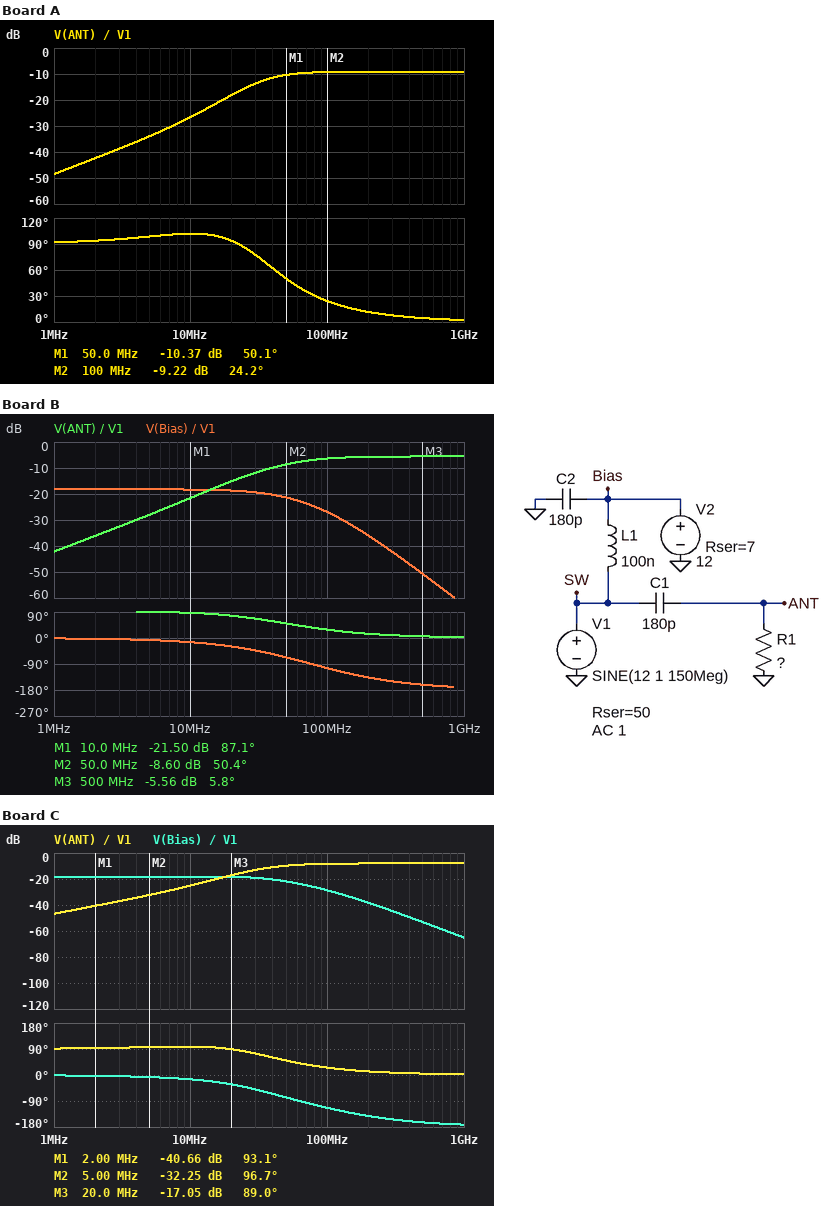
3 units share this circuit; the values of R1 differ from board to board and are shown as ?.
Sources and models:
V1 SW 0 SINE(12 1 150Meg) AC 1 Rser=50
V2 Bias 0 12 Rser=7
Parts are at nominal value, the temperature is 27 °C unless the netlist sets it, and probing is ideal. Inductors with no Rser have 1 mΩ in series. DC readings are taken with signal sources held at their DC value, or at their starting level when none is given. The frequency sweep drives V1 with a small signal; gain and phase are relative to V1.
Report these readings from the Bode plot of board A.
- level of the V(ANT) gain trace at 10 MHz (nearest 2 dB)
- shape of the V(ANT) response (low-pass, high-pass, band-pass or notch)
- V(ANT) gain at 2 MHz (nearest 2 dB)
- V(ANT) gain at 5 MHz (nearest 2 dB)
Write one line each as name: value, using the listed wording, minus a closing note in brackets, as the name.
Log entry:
level of the V(ANT) gain trace at 10 MHz: -26 dB
shape of the V(ANT) response: high-pass
V(ANT) gain at 2 MHz: -42 dB
V(ANT) gain at 5 MHz: -34 dB
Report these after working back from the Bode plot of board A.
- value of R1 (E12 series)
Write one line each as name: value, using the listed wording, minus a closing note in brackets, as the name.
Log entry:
value of R1: 27 Ω
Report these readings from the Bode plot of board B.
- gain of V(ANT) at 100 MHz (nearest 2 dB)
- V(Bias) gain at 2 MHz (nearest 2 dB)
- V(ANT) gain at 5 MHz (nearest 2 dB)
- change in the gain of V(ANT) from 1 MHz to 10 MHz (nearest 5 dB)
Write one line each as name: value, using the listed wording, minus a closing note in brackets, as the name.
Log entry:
gain of V(ANT) at 100 MHz: -6 dB
V(Bias) gain at 2 MHz: -18 dB
V(ANT) gain at 5 MHz: -28 dB
change in the gain of V(ANT) from 1 MHz to 10 MHz: 20 dB
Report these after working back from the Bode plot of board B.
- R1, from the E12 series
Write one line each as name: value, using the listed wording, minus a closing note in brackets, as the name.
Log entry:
R1, from the E12 series: 56 Ω
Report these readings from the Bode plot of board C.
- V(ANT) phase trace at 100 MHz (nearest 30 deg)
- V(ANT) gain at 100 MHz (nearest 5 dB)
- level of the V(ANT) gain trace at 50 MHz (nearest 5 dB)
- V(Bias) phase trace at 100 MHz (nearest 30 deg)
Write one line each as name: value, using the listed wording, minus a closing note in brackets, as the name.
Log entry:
V(ANT) phase trace at 100 MHz: 30 deg
V(ANT) gain at 100 MHz: -10 dB
level of the V(ANT) gain trace at 50 MHz: -10 dB
V(Bias) phase trace at 100 MHz: -120 deg
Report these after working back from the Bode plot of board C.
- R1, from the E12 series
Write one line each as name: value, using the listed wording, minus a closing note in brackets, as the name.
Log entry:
R1, from the E12 series: 33 Ω
